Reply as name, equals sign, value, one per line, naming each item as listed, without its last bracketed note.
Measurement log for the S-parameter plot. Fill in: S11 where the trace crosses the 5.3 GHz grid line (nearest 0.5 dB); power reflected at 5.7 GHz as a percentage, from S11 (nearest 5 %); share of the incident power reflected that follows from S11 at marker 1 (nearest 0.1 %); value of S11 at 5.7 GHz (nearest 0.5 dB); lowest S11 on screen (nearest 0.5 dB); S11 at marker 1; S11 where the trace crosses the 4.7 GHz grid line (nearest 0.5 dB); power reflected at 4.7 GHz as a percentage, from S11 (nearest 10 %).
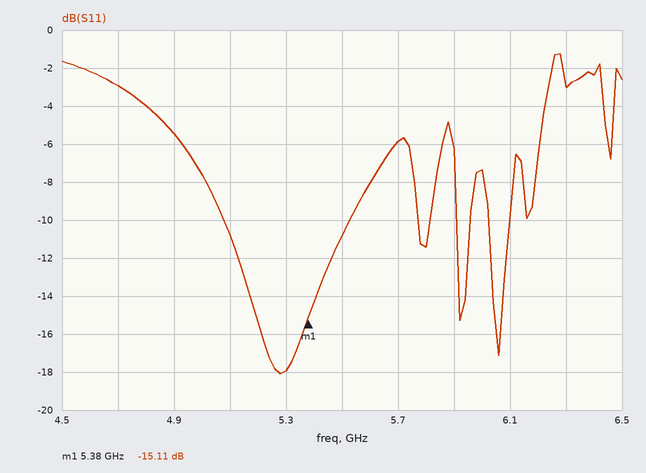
S11 where the trace crosses the 5.3 GHz grid line = -18.0 dB
power reflected at 5.7 GHz as a percentage, from S11 = 25 %
share of the incident power reflected that follows from S11 at marker 1 = 3.1 %
value of S11 at 5.7 GHz = -6.0 dB
lowest S11 on screen = -18.0 dB
S11 at marker 1 = -15.11 dB
S11 where the trace crosses the 4.7 GHz grid line = -3.0 dB
power reflected at 4.7 GHz as a percentage, from S11 = 50 %
